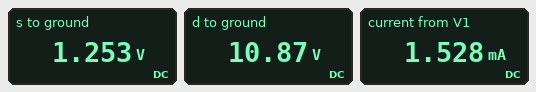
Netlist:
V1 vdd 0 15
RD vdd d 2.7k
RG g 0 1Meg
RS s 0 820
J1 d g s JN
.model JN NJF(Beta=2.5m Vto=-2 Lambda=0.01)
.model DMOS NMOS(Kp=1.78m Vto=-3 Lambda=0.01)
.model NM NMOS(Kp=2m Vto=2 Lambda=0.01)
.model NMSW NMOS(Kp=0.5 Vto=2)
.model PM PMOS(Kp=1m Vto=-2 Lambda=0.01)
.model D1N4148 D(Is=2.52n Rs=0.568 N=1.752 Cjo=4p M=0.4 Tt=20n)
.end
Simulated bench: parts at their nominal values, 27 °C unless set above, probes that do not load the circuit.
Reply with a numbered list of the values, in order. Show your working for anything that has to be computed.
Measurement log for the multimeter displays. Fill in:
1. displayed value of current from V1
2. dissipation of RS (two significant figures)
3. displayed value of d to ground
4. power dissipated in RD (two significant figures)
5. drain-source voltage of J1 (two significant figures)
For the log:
1. 1.528 mA
2. (1.253 V)^2 / 820 Ω = 1.9 mW
3. 10.87 V
4. (15 V - 10.87 V)^2 / 2.7 kΩ = 6.3 mW
5. 10.87 V - 1.253 V = 9.6 V
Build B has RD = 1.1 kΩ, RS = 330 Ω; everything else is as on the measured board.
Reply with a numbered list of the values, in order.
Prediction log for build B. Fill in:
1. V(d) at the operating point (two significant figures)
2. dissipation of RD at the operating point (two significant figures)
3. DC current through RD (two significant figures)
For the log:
1. 12 V
2. 9.5 mW
3. 2.9 mA
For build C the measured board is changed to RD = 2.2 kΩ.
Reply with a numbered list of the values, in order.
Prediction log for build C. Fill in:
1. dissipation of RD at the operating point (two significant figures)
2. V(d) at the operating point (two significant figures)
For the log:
1. 5.2 mW
2. 12 V
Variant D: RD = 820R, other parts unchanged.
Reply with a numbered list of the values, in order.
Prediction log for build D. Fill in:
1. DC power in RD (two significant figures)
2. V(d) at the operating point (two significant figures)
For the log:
1. 1.9 mW
2. 14 V
